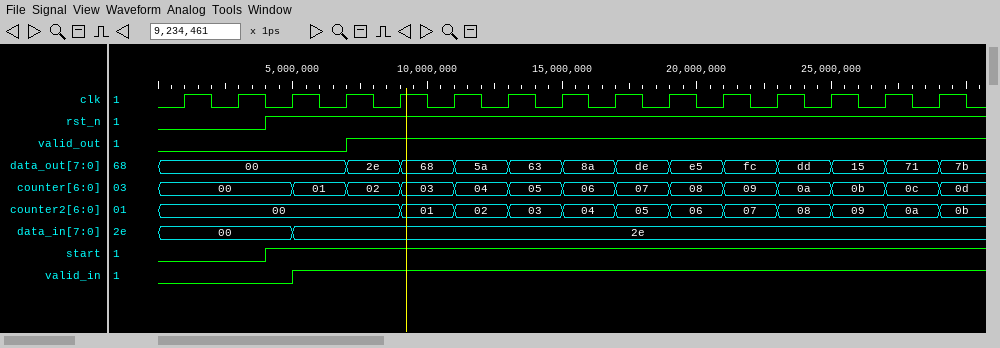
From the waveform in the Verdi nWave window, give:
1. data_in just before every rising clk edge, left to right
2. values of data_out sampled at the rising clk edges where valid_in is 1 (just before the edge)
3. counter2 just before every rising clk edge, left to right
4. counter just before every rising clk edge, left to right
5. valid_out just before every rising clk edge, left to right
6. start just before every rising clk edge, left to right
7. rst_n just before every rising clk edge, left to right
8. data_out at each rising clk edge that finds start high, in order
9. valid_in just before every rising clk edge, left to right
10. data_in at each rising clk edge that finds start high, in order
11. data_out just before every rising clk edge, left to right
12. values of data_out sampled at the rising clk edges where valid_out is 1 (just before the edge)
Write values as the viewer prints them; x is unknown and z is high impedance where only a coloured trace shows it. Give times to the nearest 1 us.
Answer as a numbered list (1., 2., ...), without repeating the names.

1. 00, 00, 00, 2e, 2e, 2e, 2e, 2e, 2e, 2e, 2e, 2e, 2e, 2e, 2e
2. 00, 2e, 68, 5a, 63, 8a, de, e5, fc, dd, 15, 71
3. 00, 00, 00, 00, 00, 01, 02, 03, 04, 05, 06, 07, 08, 09, 0a
4. 00, 00, 00, 01, 02, 03, 04, 05, 06, 07, 08, 09, 0a, 0b, 0c
5. 0 0 0 0 1 1 1 1 1 1 1 1 1 1 1
6. 0 0 1 1 1 1 1 1 1 1 1 1 1 1 1
7. 0 0 1 1 1 1 1 1 1 1 1 1 1 1 1
8. 00, 00, 2e, 68, 5a, 63, 8a, de, e5, fc, dd, 15, 71
9. 0 0 0 1 1 1 1 1 1 1 1 1 1 1 1
10. 00, 2e, 2e, 2e, 2e, 2e, 2e, 2e, 2e, 2e, 2e, 2e, 2e
11. 00, 00, 00, 00, 2e, 68, 5a, 63, 8a, de, e5, fc, dd, 15, 71
12. 2e, 68, 5a, 63, 8a, de, e5, fc, dd, 15, 71
